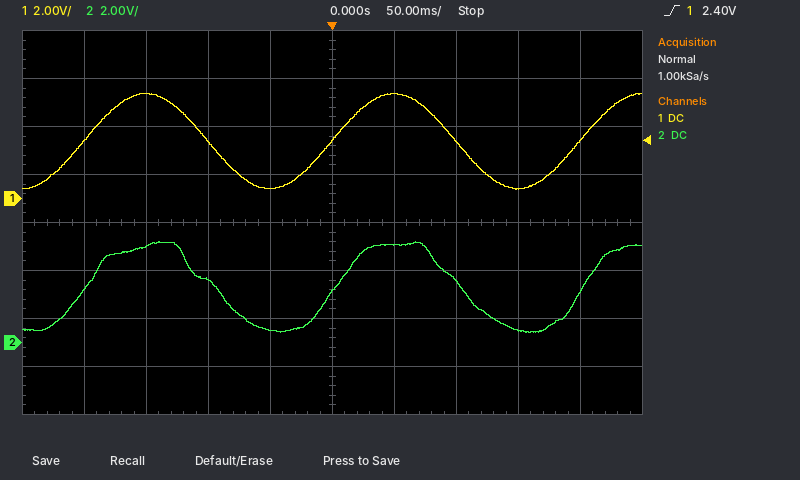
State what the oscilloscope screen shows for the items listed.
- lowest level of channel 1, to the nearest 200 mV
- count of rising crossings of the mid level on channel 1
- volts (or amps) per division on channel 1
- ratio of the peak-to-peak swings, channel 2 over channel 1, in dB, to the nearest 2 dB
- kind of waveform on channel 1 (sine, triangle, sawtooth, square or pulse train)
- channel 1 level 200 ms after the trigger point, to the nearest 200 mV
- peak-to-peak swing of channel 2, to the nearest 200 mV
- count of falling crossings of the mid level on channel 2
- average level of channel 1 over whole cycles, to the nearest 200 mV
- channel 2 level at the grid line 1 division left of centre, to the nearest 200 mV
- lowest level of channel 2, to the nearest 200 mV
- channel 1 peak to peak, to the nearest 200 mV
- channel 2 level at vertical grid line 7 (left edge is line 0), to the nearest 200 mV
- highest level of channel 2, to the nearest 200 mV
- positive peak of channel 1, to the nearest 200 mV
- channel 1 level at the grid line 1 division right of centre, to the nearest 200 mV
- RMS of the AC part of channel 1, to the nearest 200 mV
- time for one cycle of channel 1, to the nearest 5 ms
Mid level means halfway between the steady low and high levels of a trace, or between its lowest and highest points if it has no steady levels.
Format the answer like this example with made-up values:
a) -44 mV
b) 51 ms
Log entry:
a) 400 mV
b) 3
c) 2 V
d) 0 dB
e) sine
f) 2.4 V
g) 3.8 V
h) 2
i) 2.4 V
j) 600 mV
k) 400 mV
l) 4.0 V
m) 2.6 V
n) 4.2 V
o) 4.4 V
p) 4.4 V
q) 1.4 V
r) 200 ms
